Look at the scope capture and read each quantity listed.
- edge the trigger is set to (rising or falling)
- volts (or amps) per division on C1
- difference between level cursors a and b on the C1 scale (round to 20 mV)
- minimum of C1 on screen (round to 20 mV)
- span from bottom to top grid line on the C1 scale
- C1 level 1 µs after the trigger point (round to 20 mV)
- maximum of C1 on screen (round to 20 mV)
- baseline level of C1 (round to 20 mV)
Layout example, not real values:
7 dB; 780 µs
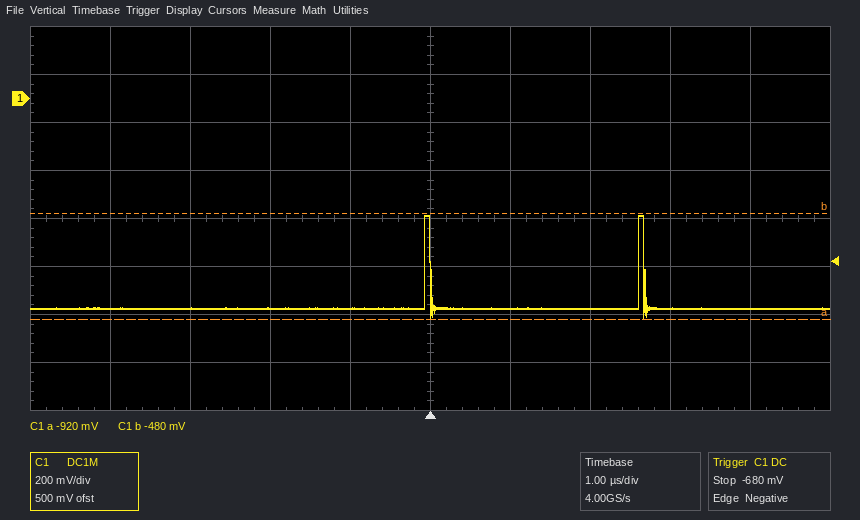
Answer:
falling; 200 mV; 440 mV; -920 mV; 1.6 V; -880 mV; -480 mV; -880 mV
